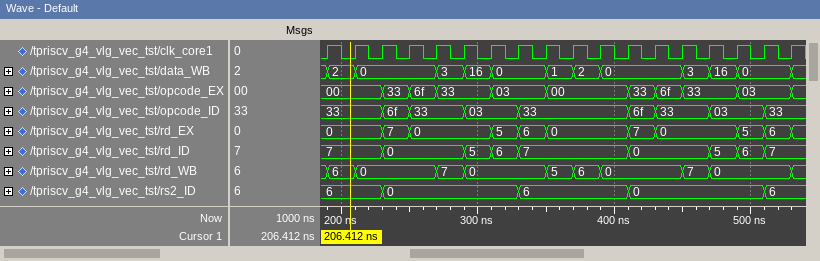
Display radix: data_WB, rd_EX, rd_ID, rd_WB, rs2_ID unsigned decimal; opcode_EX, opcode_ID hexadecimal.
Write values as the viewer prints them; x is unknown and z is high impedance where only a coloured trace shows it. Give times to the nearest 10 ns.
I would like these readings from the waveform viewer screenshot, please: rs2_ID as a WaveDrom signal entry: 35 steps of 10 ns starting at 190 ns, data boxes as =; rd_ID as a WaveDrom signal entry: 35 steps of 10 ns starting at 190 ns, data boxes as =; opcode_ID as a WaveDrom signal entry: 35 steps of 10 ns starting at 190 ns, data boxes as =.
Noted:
{name: 'rs2_ID', wave: '=...=.........=.......=.........=..', data: '6 0 6 0 6'}
{name: 'rd_ID', wave: '=...=.....=.=.=.......=.....=.=.=..', data: '7 0 5 6 7 0 5 6 7'}
{name: 'opcode_ID', wave: '=...=.=...=...=.......=.=...=...=..', data: '33 6f 33 03 33 6f 33 03 33'}
